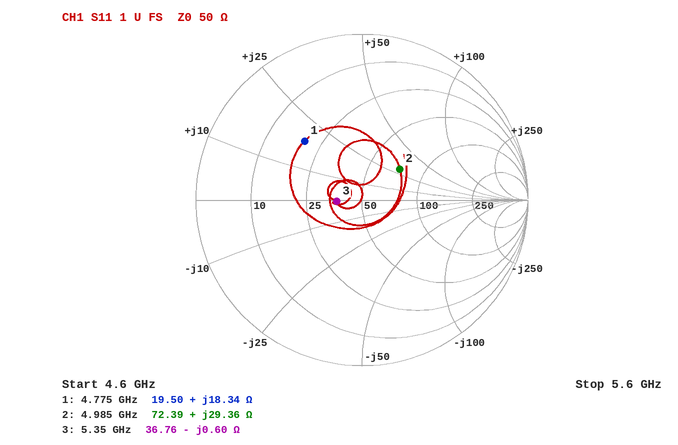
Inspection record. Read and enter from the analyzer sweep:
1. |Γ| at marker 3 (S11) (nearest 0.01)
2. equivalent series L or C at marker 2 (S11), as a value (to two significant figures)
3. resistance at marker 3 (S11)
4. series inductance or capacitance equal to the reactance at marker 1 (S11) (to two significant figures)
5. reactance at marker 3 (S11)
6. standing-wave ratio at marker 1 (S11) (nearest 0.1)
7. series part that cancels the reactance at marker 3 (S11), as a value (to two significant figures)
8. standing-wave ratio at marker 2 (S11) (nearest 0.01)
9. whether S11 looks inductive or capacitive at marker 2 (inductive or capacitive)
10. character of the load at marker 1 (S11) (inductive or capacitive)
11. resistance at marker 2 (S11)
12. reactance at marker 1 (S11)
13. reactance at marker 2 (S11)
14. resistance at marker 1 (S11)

0.15
940 pH
36.76 Ω
610 pH
-0.60 Ω
3.0
18 pH
1.83
inductive
inductive
72.39 Ω
+18.34 Ω
+29.36 Ω
19.50 Ω
